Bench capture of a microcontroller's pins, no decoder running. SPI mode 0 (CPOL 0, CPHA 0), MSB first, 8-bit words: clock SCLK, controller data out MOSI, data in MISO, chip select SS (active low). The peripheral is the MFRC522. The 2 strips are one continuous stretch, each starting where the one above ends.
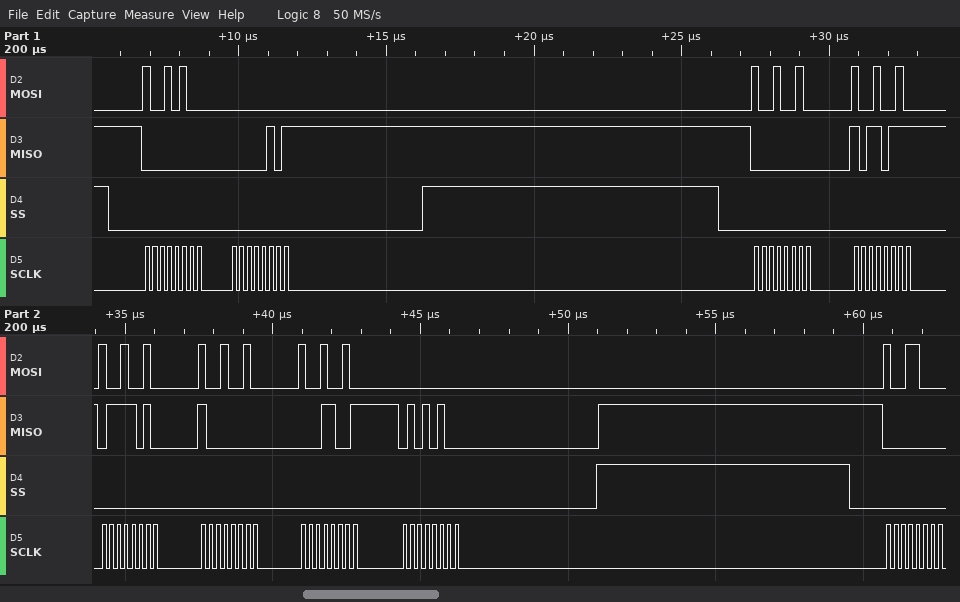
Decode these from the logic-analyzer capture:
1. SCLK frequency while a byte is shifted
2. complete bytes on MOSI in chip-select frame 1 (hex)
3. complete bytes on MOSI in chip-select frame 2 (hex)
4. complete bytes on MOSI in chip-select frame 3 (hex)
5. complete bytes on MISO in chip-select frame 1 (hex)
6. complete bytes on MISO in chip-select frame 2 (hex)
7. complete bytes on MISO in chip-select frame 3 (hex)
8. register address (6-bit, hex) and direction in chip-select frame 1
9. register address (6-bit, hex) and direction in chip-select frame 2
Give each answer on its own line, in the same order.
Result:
4 MHz
0x94 0x00
0x92 0x92 0x92 0x92 0x92 0x00
0x98
0x00 0x05
0x00 0xB7 0x7A 0x80 0x19 0x54
0x00
0x0A read
0x09 read
